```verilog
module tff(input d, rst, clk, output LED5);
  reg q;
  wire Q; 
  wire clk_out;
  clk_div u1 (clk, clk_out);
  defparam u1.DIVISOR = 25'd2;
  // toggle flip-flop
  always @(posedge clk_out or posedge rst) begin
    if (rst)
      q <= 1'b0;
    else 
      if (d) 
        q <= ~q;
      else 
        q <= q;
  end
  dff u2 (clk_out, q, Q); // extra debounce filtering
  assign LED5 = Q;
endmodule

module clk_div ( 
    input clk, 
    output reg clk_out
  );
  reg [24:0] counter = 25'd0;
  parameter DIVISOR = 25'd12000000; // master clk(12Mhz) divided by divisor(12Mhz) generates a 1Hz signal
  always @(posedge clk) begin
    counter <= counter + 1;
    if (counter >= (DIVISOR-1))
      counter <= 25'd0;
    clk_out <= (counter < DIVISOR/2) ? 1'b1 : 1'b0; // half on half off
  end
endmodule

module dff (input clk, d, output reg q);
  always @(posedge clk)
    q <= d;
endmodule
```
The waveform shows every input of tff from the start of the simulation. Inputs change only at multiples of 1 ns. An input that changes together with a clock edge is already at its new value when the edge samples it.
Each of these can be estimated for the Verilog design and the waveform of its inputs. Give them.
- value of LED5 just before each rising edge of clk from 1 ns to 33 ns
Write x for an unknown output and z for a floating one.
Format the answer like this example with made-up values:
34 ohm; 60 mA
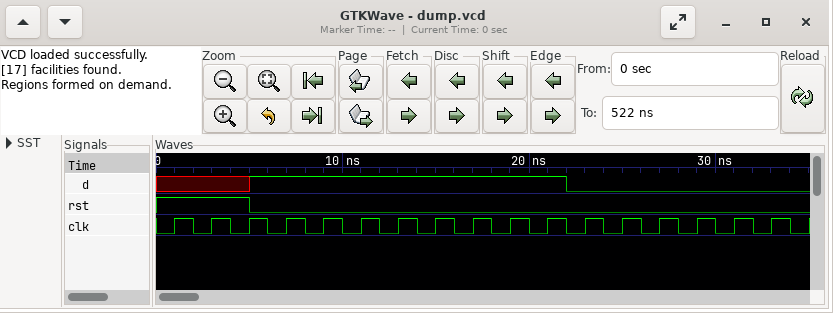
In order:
x 0 0 0 0 1 1 0 0 1 1 0 0 1 1 1 1
